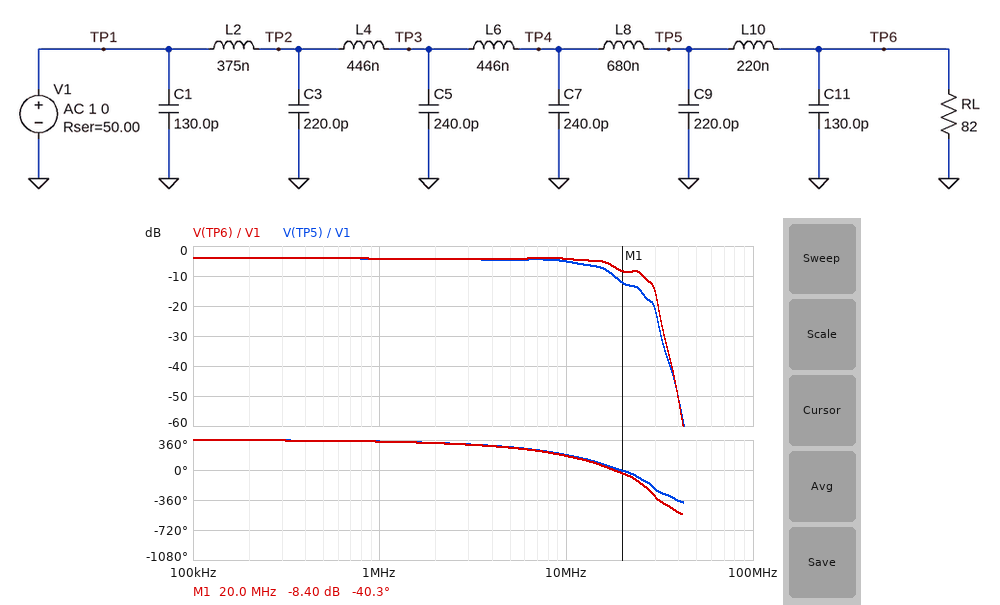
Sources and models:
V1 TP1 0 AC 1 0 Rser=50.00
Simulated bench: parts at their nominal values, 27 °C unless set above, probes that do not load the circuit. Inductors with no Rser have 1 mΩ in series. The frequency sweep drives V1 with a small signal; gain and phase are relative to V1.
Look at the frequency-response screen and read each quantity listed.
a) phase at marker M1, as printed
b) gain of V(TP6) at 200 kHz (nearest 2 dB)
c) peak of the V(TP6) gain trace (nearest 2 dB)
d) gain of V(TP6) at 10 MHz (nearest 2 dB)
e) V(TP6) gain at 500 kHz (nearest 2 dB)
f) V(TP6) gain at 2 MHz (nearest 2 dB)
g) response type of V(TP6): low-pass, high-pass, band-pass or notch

-40.3 deg
-4 dB
-4 dB
-4 dB
-4 dB
-4 dB
low-pass
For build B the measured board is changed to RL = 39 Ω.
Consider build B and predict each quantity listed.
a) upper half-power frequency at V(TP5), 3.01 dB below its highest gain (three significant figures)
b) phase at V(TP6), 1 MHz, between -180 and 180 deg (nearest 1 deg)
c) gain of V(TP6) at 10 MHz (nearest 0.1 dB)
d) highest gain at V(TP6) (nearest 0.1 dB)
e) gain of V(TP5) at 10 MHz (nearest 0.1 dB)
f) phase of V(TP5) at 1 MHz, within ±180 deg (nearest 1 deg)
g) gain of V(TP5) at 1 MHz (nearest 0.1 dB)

18.2 MHz
-18 deg
-7.6 dB
-7.1 dB
-8.0 dB
-16 deg
-7.2 dB
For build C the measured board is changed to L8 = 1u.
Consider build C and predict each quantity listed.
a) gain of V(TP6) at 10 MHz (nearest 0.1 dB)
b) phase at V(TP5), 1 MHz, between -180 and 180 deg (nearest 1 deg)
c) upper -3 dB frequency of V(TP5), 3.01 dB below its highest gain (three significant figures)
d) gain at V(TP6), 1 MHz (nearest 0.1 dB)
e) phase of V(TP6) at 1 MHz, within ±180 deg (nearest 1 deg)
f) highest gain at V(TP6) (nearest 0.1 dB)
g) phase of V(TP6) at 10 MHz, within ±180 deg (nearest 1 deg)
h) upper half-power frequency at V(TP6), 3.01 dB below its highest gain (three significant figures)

-4.7 dB
-19 deg
12.6 MHz
-4.2 dB
-20 deg
-3.9 dB
152 deg
14.8 MHz
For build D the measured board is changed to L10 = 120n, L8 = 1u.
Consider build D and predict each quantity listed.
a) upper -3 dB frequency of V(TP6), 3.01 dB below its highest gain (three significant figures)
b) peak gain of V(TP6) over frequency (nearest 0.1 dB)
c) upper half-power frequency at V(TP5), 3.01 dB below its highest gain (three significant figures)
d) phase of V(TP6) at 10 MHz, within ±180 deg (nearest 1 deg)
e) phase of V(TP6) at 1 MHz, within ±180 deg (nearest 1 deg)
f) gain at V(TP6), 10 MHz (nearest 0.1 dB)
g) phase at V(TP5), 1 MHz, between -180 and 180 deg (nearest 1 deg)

14.3 MHz
-3.9 dB
13.2 MHz
154 deg
-20 deg
-4.8 dB
-19 deg
